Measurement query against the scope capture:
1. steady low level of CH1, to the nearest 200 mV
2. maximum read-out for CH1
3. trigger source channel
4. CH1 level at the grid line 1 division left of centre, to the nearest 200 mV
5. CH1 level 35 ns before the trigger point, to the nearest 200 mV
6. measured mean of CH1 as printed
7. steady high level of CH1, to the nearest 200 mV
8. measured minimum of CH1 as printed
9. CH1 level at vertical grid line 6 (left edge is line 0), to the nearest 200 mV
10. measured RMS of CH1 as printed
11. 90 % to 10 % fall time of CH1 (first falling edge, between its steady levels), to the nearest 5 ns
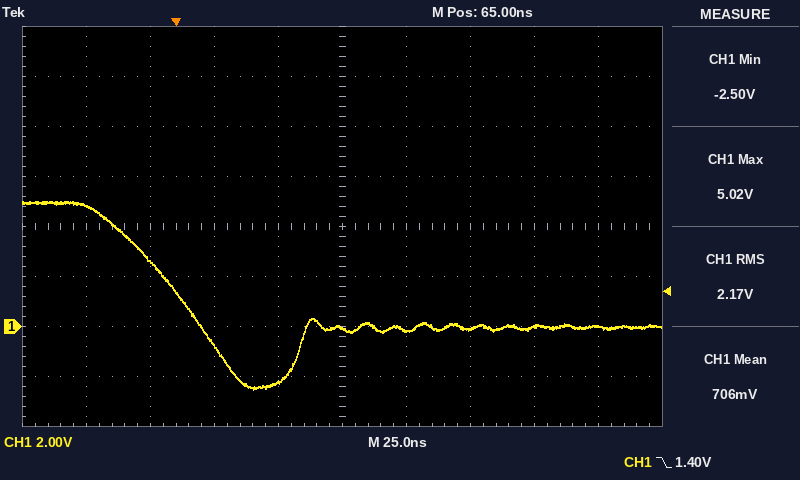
0.0 V
5.02 V
CH1
-2.2 V
4.8 V
706 mV
5.0 V
-2.50 V
-200 mV
2.17 V
35 ns
